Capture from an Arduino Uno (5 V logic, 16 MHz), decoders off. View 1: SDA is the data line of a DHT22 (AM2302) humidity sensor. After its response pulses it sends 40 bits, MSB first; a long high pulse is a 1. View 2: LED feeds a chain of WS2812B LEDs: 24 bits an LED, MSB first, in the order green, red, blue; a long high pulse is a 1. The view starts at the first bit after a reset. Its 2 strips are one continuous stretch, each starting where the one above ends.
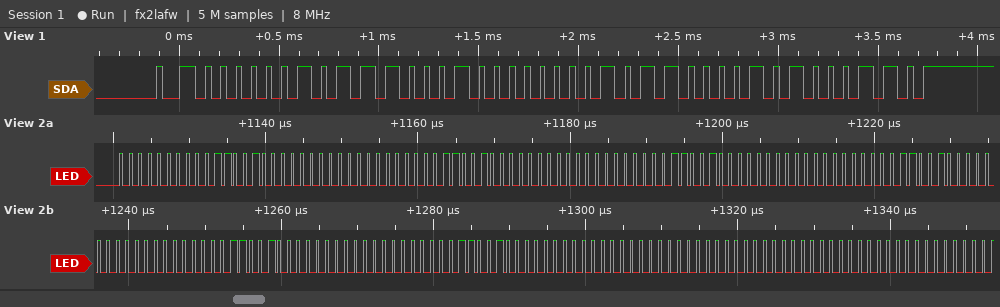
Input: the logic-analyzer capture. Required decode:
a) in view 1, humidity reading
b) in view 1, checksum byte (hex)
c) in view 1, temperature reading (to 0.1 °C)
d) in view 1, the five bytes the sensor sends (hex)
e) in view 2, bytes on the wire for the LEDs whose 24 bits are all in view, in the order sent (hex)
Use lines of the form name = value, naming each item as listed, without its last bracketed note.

in view 1, humidity reading = 73.8 %
in view 1, checksum byte = 0x46
in view 1, temperature reading = 35.3 °C
in view 1, the five bytes the sensor sends = 02 E2 01 61 46
in view 2, bytes on the wire for the LEDs whose 24 bits are all in view, in the order sent = 00 32 00 00 32 00 00 32 00 00 32 00 00 32 00 00 32 00 00 00 00
